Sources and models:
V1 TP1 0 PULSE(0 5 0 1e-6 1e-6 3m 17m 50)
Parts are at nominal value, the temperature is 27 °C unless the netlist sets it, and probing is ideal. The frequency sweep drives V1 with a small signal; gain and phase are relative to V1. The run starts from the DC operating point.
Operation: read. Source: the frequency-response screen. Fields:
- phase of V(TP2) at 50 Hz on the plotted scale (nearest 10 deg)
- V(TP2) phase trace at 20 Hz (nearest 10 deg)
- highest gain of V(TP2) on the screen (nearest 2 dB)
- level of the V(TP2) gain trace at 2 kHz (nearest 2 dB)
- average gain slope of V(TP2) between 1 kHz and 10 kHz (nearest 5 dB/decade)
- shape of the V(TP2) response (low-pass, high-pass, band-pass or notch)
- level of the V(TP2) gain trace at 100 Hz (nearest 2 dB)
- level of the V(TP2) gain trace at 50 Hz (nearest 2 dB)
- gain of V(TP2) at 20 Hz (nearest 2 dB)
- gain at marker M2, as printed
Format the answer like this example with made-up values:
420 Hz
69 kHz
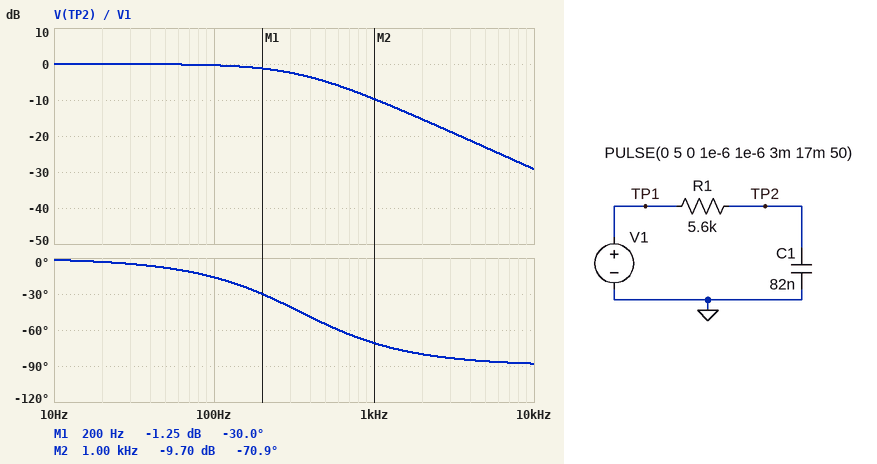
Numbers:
-10 deg
0 deg
0 dB
-16 dB
-20 dB/decade
low-pass
0 dB
0 dB
0 dB
-9.70 dB
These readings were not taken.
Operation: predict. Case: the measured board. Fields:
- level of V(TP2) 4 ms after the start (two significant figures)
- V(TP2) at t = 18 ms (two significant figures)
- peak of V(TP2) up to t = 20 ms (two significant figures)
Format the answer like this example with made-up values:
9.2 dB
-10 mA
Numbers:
570 mV
4.4 V
5.0 V
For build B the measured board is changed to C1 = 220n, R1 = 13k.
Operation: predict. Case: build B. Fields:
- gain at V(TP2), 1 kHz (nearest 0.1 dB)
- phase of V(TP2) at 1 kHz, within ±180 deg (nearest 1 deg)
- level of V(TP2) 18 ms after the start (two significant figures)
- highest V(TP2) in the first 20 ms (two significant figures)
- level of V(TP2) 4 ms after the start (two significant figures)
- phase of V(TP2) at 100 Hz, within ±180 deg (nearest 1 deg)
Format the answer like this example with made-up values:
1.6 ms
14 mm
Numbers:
-25.1 dB
-87 deg
1.5 V
3.3 V
2.3 V
-61 deg
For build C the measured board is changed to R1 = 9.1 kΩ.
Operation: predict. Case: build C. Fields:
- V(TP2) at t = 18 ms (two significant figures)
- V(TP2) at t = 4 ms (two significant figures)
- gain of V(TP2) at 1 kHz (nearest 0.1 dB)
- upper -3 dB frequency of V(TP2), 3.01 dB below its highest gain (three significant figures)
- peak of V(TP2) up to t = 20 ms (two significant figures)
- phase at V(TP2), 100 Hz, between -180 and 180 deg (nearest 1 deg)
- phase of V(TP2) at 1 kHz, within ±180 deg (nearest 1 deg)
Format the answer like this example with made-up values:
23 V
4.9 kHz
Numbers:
3.7 V
1.3 V
-13.6 dB
213 Hz
4.9 V
-25 deg
-78 deg
